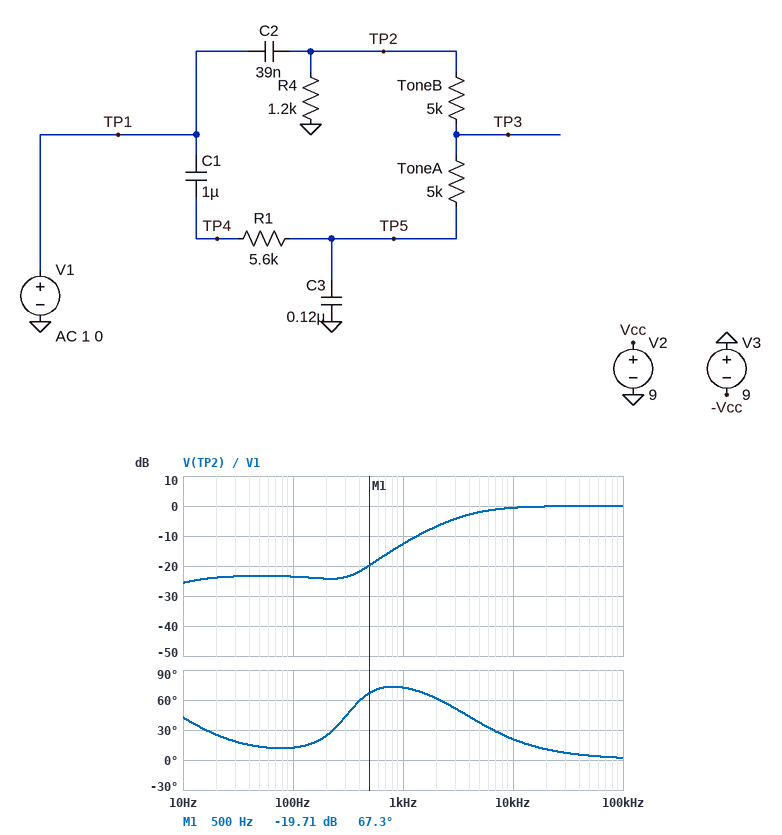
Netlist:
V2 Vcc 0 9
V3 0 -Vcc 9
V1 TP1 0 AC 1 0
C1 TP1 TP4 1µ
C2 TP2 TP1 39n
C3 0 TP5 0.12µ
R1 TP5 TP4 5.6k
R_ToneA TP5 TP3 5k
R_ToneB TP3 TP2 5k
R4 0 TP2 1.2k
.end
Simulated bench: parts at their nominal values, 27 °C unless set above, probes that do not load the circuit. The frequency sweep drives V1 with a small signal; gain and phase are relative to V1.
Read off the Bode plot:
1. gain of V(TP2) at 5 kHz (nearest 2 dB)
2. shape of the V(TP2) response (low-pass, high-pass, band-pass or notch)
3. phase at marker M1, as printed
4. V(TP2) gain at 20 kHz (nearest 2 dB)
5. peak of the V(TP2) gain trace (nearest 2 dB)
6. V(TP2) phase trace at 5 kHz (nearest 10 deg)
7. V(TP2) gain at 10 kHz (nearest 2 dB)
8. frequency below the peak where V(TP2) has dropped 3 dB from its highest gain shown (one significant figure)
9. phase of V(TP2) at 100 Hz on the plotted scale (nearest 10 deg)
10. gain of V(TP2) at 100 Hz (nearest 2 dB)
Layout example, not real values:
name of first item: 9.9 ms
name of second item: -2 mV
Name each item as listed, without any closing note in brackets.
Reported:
gain of V(TP2) at 5 kHz: -2 dB
shape of the V(TP2) response: high-pass
phase at marker M1, as printed: 67.3 deg
V(TP2) gain at 20 kHz: 0 dB
peak of the V(TP2) gain trace: 0 dB
V(TP2) phase trace at 5 kHz: 40 deg
V(TP2) gain at 10 kHz: 0 dB
frequency below the peak where V(TP2) has dropped 3 dB from its highest gain shown: 4 kHz
phase of V(TP2) at 100 Hz on the plotted scale: 10 deg
gain of V(TP2) at 100 Hz: -24 dB
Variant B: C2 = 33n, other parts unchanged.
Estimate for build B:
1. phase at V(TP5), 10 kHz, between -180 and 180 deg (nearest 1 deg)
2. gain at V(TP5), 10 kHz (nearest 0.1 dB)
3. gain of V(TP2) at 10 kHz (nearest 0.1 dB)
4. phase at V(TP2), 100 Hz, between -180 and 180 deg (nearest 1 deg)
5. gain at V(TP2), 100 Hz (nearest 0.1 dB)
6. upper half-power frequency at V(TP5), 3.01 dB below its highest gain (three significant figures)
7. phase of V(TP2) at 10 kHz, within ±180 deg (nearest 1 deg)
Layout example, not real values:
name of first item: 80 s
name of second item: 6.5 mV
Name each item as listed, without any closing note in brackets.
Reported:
phase at V(TP5), 10 kHz, between -180 and 180 deg: -80 deg
gain at V(TP5), 10 kHz: -29.1 dB
gain of V(TP2) at 10 kHz: -0.8 dB
phase at V(TP2), 100 Hz, between -180 and 180 deg: 9 deg
gain at V(TP2), 100 Hz: -23.7 dB
upper half-power frequency at V(TP5), 3.01 dB below its highest gain: 395 Hz
phase of V(TP2) at 10 kHz, within ±180 deg: 24 deg
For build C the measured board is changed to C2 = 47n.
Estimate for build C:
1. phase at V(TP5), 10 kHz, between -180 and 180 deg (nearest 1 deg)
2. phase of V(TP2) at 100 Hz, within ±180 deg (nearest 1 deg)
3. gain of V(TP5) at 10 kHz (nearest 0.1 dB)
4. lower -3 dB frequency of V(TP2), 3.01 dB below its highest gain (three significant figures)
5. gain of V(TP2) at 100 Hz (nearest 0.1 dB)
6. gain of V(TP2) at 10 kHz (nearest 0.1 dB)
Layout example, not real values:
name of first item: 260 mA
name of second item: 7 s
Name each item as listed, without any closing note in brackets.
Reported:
phase at V(TP5), 10 kHz, between -180 and 180 deg: -82 deg
phase of V(TP2) at 100 Hz, within ±180 deg: 17 deg
gain of V(TP5) at 10 kHz: -28.9 dB
lower -3 dB frequency of V(TP2), 3.01 dB below its highest gain: 3.22 kHz
gain of V(TP2) at 100 Hz: -23.3 dB
gain of V(TP2) at 10 kHz: -0.4 dB
